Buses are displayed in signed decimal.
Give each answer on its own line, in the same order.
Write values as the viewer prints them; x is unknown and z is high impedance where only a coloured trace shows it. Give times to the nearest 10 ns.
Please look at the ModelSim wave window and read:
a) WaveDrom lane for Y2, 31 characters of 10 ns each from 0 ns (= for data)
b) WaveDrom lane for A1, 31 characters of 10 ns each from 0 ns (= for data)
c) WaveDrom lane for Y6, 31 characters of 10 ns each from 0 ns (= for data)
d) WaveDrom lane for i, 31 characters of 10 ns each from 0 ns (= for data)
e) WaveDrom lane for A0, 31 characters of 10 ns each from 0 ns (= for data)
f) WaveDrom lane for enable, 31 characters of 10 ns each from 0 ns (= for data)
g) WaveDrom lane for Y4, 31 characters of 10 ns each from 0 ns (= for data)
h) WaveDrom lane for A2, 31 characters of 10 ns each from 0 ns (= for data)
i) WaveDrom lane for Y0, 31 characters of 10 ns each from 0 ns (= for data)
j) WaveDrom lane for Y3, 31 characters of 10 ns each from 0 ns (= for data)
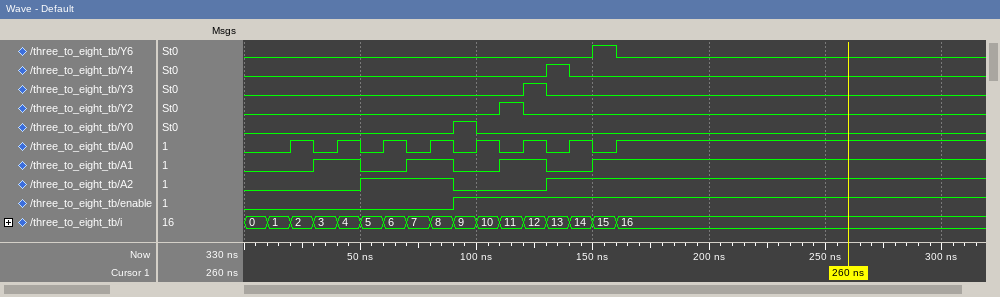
{name: 'Y2', wave: '0..........10..................'}
{name: 'A1', wave: '0..1.0.1.0.1.0.1...............'}
{name: 'Y6', wave: '0..............10..............'}
{name: 'i', wave: '=================..............', data: '0 1 2 3 4 5 6 7 8 9 10 11 12 13 14 15 16'}
{name: 'A0', wave: '0.101010101010101..............'}
{name: 'enable', wave: '0........1.....................'}
{name: 'Y4', wave: '0............10................'}
{name: 'A2', wave: '0....1...0...1.................'}
{name: 'Y0', wave: '0........10....................'}
{name: 'Y3', wave: '0...........10.................'}
